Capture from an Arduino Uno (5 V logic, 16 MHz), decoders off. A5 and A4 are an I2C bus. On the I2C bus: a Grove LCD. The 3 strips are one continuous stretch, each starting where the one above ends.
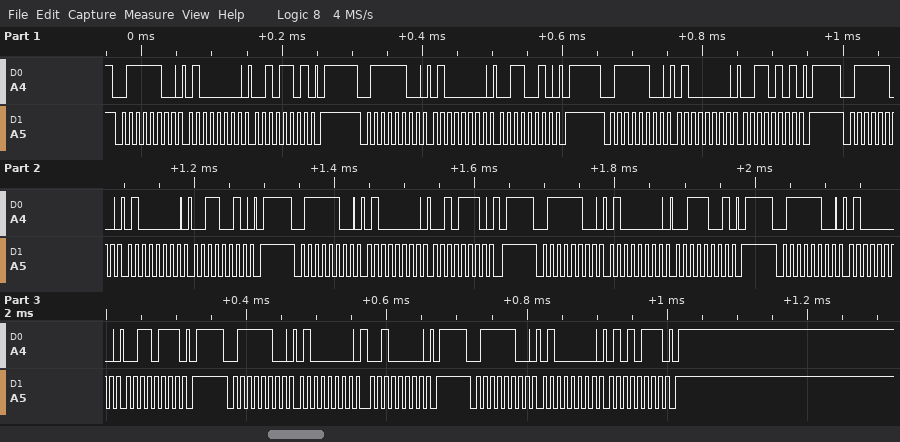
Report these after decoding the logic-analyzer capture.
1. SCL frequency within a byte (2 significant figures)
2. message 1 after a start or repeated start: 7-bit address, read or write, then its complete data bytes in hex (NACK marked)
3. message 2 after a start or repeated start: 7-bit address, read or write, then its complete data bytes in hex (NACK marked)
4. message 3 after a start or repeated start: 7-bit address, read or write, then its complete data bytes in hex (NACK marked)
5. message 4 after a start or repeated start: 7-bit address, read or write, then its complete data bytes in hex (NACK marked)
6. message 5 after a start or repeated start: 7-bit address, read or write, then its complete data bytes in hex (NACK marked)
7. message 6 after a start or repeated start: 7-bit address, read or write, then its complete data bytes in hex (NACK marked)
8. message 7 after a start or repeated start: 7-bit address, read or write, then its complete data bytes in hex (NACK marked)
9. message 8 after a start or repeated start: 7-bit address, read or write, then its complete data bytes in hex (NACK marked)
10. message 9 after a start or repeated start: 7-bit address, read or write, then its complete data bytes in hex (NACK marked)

100 kHz
0x3E write: 40 2D
0x3E write: 40 32
0x3E write: 40 35
0x3E write: 40 32
0x3E write: 40 2E
0x3E write: 40 39
0x3E write: 40 37
0x3E write: 40 20
0x3E write: 40 57
